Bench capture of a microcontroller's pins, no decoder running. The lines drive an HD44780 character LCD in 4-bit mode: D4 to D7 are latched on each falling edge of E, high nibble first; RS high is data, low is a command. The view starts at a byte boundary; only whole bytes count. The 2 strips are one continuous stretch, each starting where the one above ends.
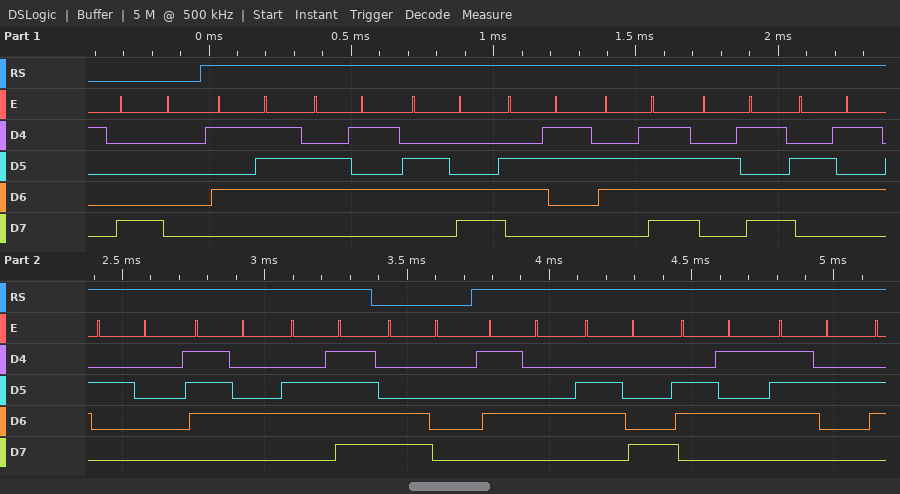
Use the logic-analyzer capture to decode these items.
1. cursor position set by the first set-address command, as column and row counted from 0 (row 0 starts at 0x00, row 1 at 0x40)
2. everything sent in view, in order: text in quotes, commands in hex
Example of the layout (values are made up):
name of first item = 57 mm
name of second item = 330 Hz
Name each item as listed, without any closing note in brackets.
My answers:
cursor position set by the first set-address command, as column and row counted from 0 = column 0, row 0
everything sent in view, in order: text in quotes, commands in hex = 0x80 "Welcome to" 0xC0 "Ther"
